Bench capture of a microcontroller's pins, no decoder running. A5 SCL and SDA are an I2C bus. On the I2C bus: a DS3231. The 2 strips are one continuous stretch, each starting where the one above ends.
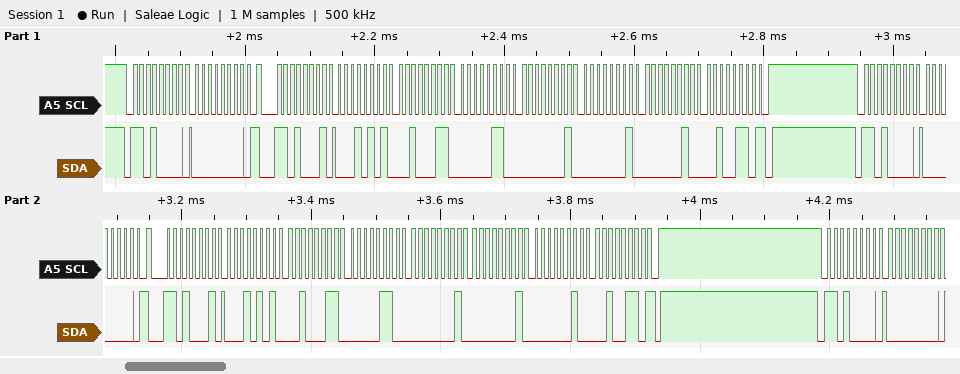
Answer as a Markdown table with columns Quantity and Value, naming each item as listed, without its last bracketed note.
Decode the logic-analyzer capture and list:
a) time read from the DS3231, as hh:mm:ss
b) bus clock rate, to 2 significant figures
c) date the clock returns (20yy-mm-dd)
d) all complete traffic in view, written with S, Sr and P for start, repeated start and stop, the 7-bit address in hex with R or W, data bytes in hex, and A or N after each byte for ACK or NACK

| Quantity | Value |
|---|---|
| time read from the DS3231, as hh:mm:ss | 06:23:15 |
| bus clock rate, to 2 significant figures | 100 kHz |
| date the clock returns | 2026-02-01 |
| all complete traffic in view, written with S, Sr and P for start, repeated start and stop, the 7-bit address in hex with R or W, data bytes in hex, and A or N after each byte for ACK or NACK | S 68W A 00 A Sr 68R A 15 A 23 A 06 A 01 A 01 A 02 A 26 N P S 68W A 00 A Sr 68R A 15 A 23 A 06 A 01 A 01 A 02 A 26 N P S 68W A 00 A |
